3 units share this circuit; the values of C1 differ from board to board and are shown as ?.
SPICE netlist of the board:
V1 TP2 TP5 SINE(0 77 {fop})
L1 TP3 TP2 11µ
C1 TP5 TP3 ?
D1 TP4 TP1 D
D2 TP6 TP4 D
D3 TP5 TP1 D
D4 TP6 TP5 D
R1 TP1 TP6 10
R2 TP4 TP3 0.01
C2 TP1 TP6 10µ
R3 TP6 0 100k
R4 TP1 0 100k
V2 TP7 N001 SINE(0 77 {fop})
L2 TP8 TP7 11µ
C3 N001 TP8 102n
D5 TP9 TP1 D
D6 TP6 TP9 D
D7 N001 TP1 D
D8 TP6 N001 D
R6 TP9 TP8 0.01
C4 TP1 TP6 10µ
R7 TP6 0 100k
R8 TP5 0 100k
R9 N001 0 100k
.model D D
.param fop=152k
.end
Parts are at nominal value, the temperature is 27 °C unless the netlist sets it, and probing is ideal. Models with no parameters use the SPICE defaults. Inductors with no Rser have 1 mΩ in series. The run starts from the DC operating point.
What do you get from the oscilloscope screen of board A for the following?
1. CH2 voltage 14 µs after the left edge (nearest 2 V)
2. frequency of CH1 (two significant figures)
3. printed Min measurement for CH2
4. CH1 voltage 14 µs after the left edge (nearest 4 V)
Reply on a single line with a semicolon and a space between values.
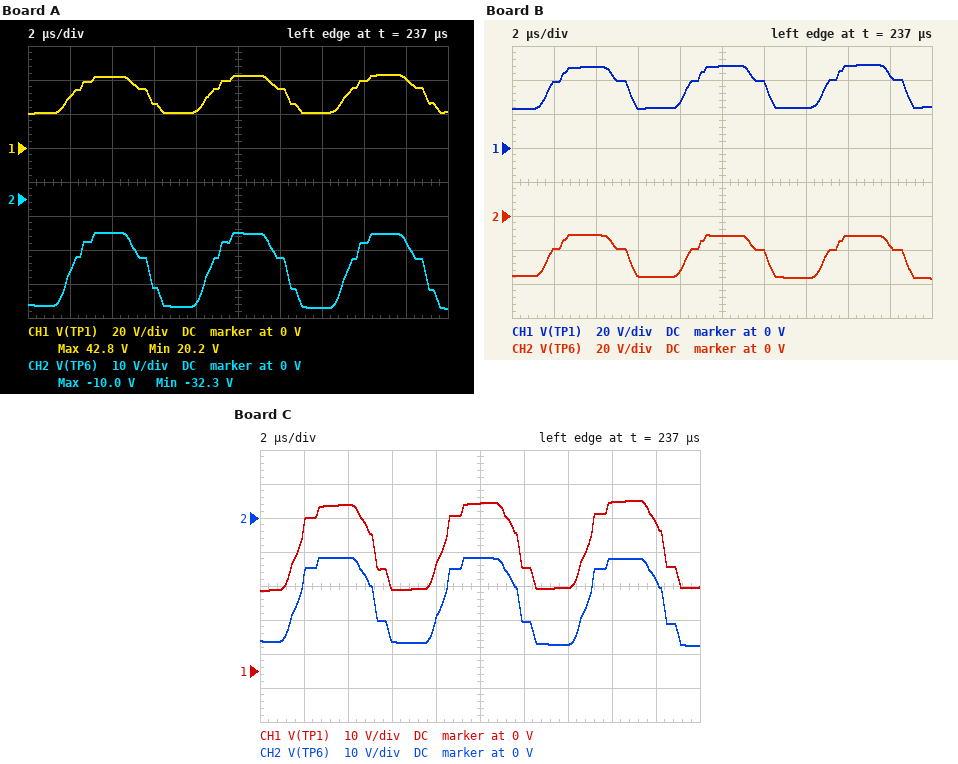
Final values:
-32 V; 150 kHz; -32.3 V; 20 V
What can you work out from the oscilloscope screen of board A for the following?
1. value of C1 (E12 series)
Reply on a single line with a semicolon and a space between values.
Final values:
150 nF
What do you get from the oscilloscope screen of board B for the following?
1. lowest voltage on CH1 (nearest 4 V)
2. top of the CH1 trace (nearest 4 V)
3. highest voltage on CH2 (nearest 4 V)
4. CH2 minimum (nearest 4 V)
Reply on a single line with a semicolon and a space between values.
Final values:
24 V; 48 V; -12 V; -36 V
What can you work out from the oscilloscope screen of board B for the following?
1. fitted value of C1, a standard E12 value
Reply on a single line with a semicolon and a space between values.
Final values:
82 nF
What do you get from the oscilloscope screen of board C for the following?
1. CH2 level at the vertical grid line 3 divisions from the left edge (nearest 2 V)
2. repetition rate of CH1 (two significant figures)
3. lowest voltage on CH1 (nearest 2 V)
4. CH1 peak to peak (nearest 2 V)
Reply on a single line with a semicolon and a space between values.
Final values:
-36 V; 150 kHz; 24 V; 26 V
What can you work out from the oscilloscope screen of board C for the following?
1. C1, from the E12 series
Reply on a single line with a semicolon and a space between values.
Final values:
56 nF
